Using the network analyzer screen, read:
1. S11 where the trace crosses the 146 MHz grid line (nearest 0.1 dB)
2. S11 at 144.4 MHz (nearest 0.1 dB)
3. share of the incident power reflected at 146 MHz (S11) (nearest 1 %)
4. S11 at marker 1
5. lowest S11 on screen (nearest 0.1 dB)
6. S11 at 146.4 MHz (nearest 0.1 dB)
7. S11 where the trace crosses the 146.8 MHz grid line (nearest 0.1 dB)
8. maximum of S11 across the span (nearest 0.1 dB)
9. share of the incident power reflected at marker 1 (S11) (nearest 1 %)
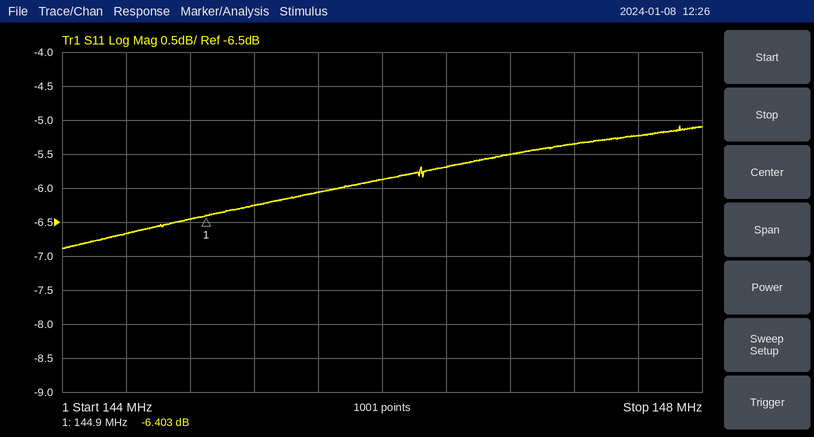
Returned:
-5.9 dB
-6.7 dB
26 %
-6.403 dB
-6.9 dB
-5.7 dB
-5.5 dB
-5.1 dB
23 %
